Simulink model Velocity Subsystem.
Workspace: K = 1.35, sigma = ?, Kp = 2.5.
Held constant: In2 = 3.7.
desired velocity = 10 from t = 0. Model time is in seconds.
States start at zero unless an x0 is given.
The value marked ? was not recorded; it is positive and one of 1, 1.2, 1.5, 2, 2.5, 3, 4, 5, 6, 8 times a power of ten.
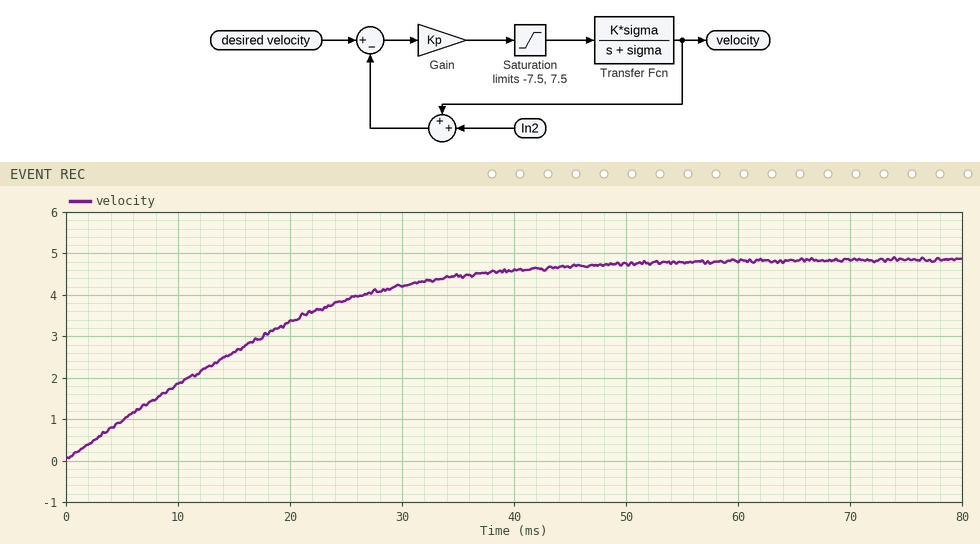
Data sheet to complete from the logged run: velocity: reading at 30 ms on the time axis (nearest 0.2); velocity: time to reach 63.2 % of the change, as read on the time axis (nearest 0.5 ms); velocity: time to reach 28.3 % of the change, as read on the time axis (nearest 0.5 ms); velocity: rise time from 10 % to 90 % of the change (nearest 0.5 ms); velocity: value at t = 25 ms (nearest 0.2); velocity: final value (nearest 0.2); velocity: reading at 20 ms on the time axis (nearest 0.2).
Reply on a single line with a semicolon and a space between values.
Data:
4.2; 18.0 ms; 7.5 ms; 30.5 ms; 3.8; 4.8; 3.4
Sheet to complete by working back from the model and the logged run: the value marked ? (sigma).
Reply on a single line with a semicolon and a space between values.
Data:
20
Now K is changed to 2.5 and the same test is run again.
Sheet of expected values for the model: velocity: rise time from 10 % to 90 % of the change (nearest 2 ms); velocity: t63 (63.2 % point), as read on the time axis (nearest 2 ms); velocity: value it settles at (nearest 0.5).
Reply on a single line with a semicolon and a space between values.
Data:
18 ms; 10 ms; 5.5
